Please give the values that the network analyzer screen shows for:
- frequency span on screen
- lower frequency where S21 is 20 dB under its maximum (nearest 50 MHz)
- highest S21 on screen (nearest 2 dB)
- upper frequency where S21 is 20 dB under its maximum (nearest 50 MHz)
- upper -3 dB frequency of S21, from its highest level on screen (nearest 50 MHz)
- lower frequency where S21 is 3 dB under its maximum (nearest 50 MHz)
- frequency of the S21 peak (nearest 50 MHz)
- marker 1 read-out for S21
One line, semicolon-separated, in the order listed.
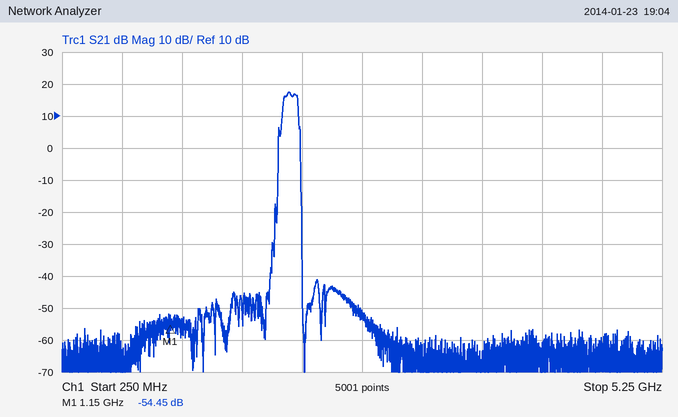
5 GHz; 2.05 GHz; 18 dB; 2.25 GHz; 2.20 GHz; 2.10 GHz; 2.15 GHz; -54.45 dB
